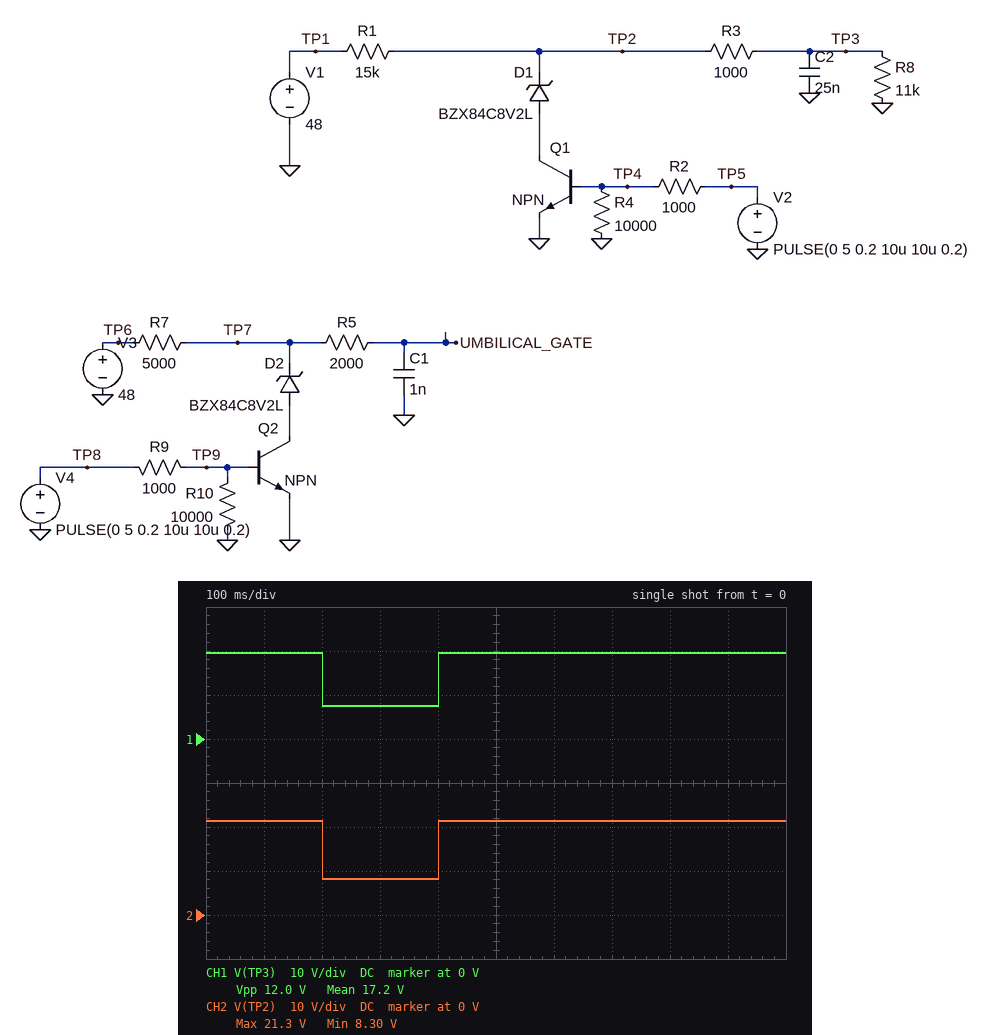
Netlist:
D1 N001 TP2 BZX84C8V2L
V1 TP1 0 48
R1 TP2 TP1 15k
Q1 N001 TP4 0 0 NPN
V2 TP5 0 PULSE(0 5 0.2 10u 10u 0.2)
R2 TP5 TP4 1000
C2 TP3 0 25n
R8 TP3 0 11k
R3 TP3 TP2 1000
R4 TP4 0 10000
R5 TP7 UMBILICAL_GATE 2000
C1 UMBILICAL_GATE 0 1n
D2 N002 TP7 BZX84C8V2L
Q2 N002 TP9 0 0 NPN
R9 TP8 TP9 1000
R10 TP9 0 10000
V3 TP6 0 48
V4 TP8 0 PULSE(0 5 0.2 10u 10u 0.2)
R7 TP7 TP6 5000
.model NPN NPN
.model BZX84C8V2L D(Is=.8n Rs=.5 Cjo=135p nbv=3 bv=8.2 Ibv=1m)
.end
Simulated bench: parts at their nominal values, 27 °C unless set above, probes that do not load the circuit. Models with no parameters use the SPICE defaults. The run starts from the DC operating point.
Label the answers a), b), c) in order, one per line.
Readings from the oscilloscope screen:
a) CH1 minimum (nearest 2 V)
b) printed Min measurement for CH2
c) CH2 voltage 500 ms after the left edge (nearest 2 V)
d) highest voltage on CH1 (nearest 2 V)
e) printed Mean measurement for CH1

a) 8 V
b) 8.30 V
c) 22 V
d) 20 V
e) 17.2 V
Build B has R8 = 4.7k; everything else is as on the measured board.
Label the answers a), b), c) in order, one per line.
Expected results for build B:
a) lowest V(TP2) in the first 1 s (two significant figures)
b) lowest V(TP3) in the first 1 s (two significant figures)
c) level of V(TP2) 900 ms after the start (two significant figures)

a) 8.2 V
b) 6.8 V
c) 13 V
